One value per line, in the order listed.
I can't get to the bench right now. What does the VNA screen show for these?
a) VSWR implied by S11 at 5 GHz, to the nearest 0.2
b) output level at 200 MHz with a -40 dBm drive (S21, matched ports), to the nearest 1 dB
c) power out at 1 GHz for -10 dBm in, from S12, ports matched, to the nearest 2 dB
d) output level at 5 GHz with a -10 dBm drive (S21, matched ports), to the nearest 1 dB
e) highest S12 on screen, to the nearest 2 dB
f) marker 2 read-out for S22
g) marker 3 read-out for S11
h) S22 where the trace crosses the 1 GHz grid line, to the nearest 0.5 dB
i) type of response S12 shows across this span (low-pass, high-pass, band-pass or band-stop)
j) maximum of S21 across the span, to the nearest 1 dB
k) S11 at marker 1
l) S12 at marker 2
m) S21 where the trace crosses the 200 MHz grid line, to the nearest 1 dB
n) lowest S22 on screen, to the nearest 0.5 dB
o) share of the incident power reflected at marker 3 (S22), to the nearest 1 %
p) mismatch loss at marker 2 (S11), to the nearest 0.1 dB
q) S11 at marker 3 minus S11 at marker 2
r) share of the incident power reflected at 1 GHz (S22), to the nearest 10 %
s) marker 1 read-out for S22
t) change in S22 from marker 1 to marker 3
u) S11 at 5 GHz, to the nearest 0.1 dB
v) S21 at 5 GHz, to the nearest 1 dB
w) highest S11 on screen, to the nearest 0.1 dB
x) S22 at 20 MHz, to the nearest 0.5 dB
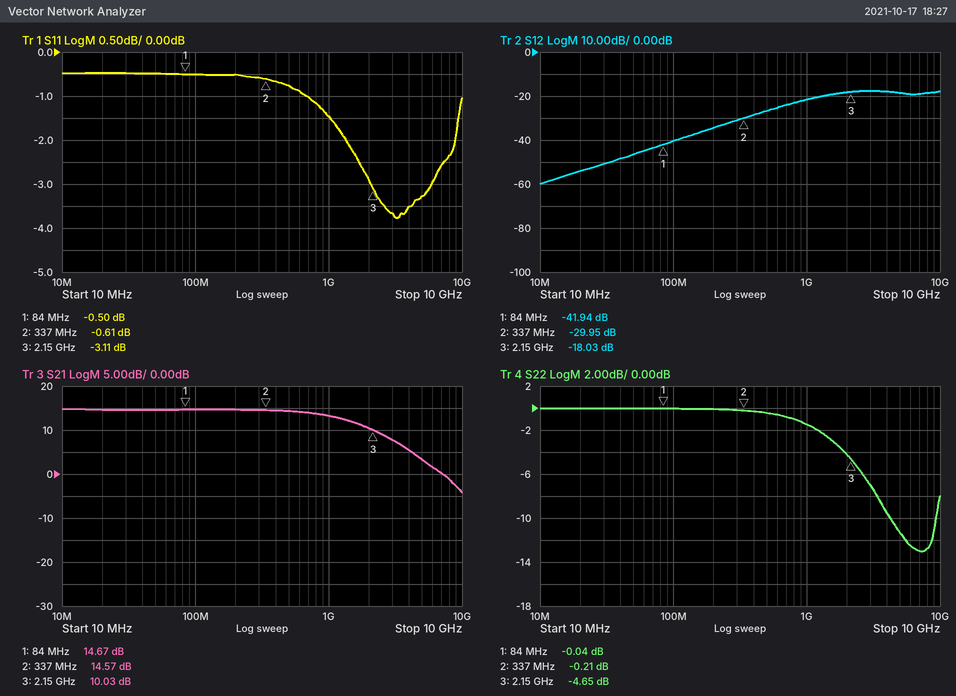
5.4
-25 dBm
-32 dBm
-7 dBm
-18 dB
-0.21 dB
-3.11 dB
-1.5 dB
high-pass
15 dB
-0.50 dB
-29.95 dB
15 dB
-13.0 dB
34 %
8.8 dB
-2.50 dB
70 %
-0.04 dB
-4.61 dB
-3.3 dB
3 dB
-0.5 dB
0.0 dB
